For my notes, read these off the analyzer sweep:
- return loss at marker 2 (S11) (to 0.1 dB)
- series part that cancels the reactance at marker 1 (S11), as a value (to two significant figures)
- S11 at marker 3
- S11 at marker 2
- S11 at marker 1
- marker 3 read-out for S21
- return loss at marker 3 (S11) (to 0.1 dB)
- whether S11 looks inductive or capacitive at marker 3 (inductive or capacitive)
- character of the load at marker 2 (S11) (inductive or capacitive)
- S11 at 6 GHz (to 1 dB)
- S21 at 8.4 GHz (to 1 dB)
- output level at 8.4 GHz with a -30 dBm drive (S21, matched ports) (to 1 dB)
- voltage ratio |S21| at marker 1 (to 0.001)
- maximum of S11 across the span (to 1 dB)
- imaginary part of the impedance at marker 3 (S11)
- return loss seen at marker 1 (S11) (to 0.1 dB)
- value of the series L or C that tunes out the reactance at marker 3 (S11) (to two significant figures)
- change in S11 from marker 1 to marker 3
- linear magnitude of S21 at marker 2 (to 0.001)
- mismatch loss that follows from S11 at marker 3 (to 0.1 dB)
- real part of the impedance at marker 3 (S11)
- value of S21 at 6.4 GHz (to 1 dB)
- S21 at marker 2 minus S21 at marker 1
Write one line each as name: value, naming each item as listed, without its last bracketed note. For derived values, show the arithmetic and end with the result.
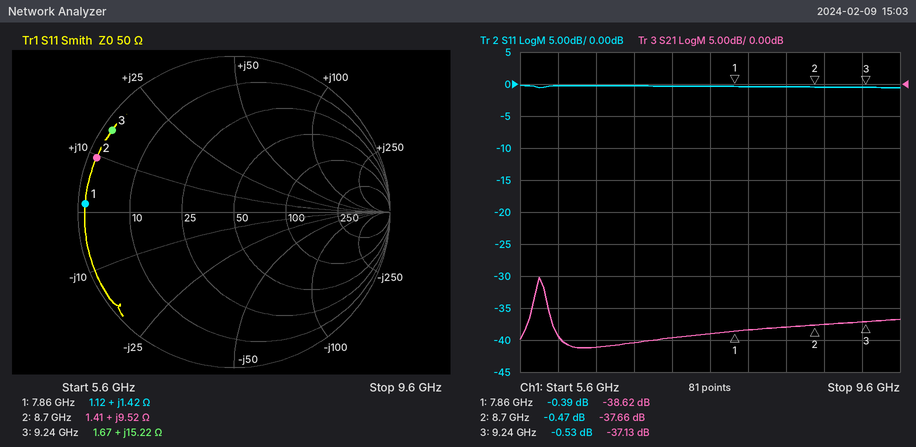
return loss at marker 2 (S11): 0.5 dB
series part that cancels the reactance at marker 1 (S11), as a value: C = 1/(2π × 7.86 GHz × 1.42 Ω) ≈ 14 pF
S11 at marker 3: -0.53 dB
S11 at marker 2: -0.47 dB
S11 at marker 1: -0.39 dB
marker 3 read-out for S21: -37.13 dB
return loss at marker 3 (S11): 0.5 dB
whether S11 looks inductive or capacitive at marker 3: inductive
character of the load at marker 2 (S11): inductive
S11 at 6 GHz: 0 dB
S21 at 8.4 GHz: -38 dB
output level at 8.4 GHz with a -30 dBm drive (S21, matched ports): -30 dBm + (-38 dB) = -68 dBm
voltage ratio |S21| at marker 1: 10^(-38.62/20) ≈ 0.012
maximum of S11 across the span: 0 dB
imaginary part of the impedance at marker 3: +15.22 Ω
return loss seen at marker 1 (S11): 0.4 dB
value of the series L or C that tunes out the reactance at marker 3 (S11): C = 1/(2π × 9.24 GHz × 15.22 Ω) ≈ 1.1 pF
change in S11 from marker 1 to marker 3: -0.53 − (-0.39) = -0.14 dB
linear magnitude of S21 at marker 2: 10^(-37.66/20) ≈ 0.013
mismatch loss that follows from S11 at marker 3: −10 log10(1 − 10^(-0.53/10)) ≈ 9.4 dB
real part of the impedance at marker 3: 1.67 Ω
value of S21 at 6.4 GHz: -41 dB
S21 at marker 2 minus S21 at marker 1: -37.66 − (-38.62) = 0.96 dB
